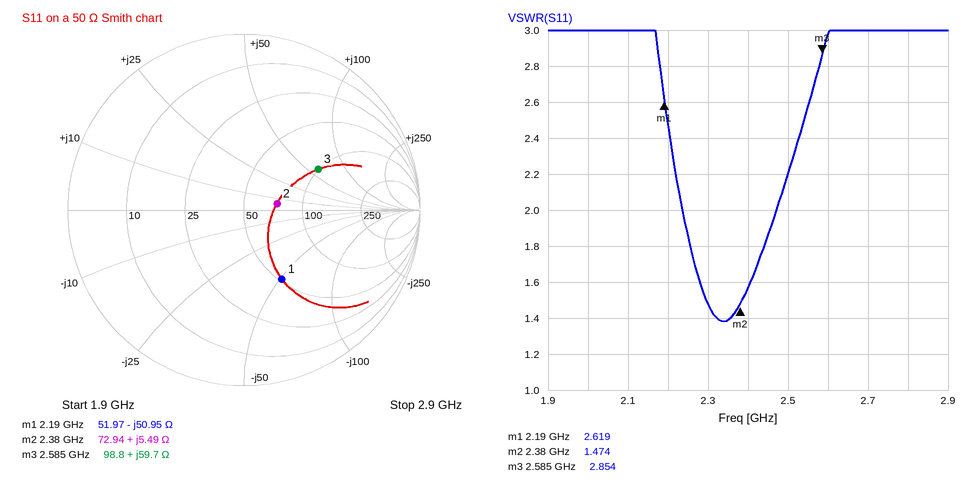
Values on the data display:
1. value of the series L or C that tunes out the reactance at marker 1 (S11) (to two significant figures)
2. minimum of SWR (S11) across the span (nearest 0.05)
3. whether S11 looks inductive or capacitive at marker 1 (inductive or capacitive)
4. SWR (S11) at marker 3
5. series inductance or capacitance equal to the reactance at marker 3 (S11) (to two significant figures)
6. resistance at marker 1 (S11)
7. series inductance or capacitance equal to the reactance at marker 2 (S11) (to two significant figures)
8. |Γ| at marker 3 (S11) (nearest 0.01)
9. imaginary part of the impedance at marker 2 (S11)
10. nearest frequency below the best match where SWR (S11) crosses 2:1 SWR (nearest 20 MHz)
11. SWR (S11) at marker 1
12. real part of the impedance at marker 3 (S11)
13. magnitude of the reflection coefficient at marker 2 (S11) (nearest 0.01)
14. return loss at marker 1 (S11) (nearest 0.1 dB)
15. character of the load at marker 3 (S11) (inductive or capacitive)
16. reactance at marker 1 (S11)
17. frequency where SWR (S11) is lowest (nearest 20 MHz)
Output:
3.7 nH
1.40
capacitive
2.854
3.7 nH
51.97 Ω
370 pH
0.48
+5.49 Ω
2.24 GHz
2.619
98.8 Ω
0.19
7.0 dB
inductive
-50.95 Ω
2.34 GHz
